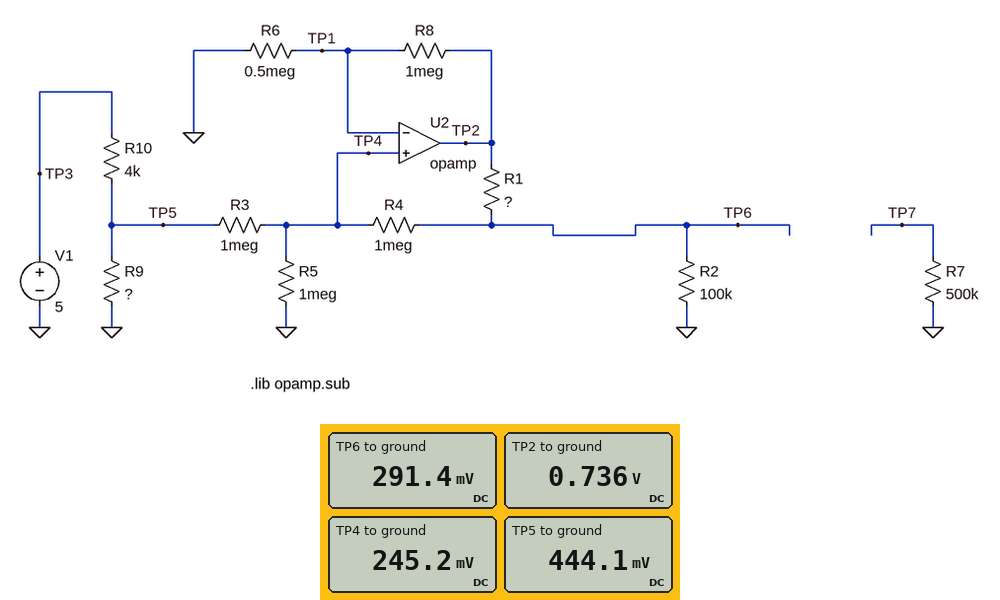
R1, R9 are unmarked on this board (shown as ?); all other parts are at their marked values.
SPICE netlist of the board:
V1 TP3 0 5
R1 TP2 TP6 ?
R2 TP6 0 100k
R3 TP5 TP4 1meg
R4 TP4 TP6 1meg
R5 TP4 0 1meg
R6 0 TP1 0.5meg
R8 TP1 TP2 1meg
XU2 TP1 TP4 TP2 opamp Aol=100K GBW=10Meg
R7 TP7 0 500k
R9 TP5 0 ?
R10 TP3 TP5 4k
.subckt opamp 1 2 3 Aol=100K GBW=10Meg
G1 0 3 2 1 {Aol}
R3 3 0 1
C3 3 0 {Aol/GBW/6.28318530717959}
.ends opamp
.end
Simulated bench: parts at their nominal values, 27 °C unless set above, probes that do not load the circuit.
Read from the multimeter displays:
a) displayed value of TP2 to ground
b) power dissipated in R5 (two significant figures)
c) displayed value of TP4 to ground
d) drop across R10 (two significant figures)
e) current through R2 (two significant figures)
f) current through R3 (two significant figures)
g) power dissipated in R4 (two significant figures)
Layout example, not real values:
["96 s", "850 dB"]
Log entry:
["0.736 V", "60 nW", "245.2 mV", "4.6 V", "2.9 µA", "200 nA", "2.1 nW"]
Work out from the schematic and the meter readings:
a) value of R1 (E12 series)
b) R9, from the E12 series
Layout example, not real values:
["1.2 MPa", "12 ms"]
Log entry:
["150 kΩ", "390 Ω"]
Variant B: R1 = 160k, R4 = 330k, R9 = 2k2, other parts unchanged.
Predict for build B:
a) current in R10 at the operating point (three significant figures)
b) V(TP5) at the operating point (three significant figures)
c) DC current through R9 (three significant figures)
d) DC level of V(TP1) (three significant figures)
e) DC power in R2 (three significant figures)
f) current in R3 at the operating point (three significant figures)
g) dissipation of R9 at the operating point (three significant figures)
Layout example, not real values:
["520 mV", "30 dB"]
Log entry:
["807 µA", "1.77 V", "806 µA", "1.10 V", "15.5 µW", "670 nA", "1.43 mW"]
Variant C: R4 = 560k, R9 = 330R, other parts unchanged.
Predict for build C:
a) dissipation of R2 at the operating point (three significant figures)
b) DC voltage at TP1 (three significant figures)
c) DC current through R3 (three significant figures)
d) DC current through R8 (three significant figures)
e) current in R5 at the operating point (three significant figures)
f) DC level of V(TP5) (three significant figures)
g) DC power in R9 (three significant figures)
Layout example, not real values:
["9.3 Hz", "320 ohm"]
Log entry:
["719 nW", "227 mV", "154 nA", "454 nA", "227 nA", "381 mV", "440 µW"]
